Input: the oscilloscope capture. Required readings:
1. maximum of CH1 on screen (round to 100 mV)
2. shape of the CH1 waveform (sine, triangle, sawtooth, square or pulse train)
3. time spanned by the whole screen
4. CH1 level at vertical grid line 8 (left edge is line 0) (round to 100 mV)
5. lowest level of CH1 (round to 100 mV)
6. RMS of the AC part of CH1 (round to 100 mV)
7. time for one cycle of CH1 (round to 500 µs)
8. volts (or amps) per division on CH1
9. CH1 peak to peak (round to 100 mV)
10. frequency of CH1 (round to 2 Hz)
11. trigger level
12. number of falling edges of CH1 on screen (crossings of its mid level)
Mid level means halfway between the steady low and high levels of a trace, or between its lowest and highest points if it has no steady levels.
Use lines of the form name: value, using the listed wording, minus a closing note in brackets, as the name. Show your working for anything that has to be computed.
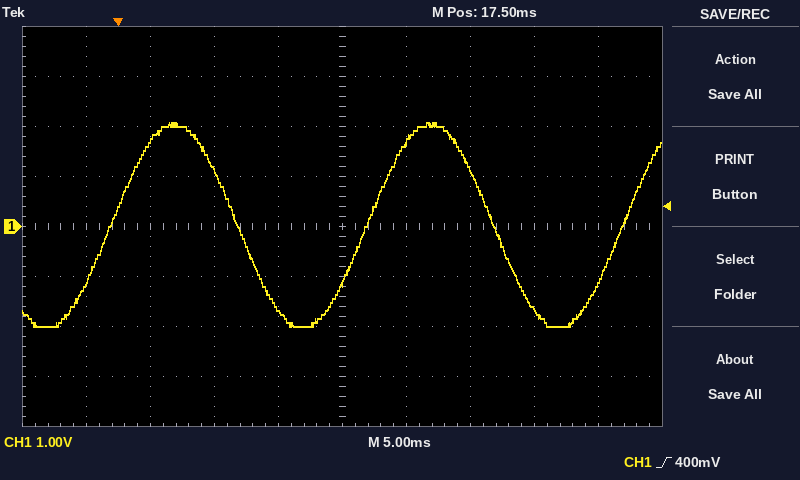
maximum of CH1 on screen: 2.1 V
shape of the CH1 waveform: sine
time spanned by the whole screen: 50 ms
CH1 level at vertical grid line 8 (left edge is line 0): -1.7 V
lowest level of CH1: -2.0 V
RMS of the AC part of CH1: 4.1 V / (2√2) ≈ 1.4 V
time for one cycle of CH1: 20.0 ms
volts (or amps) per division on CH1: 1 V
CH1 peak to peak: 2.1 V − (-2.0 V) = 4.1 V
frequency of CH1: 1 / 20.0 ms ≈ 50 Hz
trigger level: 400 mV
number of falling edges of CH1 on screen: 2
